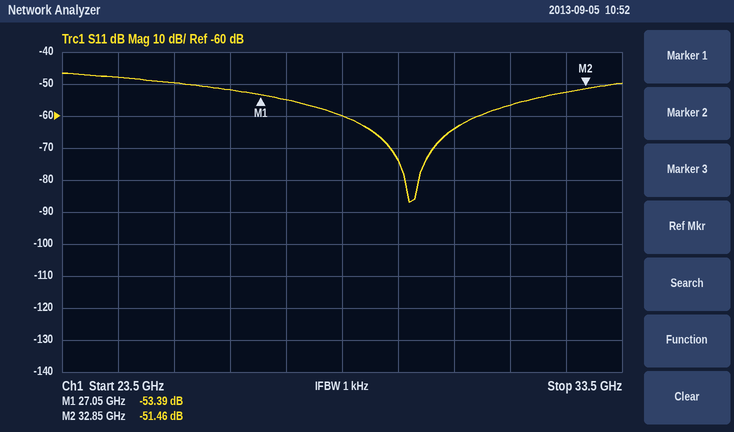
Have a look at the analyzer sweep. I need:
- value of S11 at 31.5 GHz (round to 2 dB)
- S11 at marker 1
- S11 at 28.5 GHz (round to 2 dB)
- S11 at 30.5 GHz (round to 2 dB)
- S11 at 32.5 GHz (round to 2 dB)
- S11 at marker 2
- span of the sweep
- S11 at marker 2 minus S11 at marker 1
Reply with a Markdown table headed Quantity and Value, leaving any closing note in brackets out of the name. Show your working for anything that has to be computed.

| Quantity | Value |
|---|---|
| value of S11 at 31.5 GHz | -56 dB |
| S11 at marker 1 | -53.39 dB |
| S11 at 28.5 GHz | -60 dB |
| S11 at 30.5 GHz | -64 dB |
| S11 at 32.5 GHz | -52 dB |
| S11 at marker 2 | -51.46 dB |
| span of the sweep | 10 GHz |
| S11 at marker 2 minus S11 at marker 1 | -51.46 − (-53.39) = 1.93 dB |
